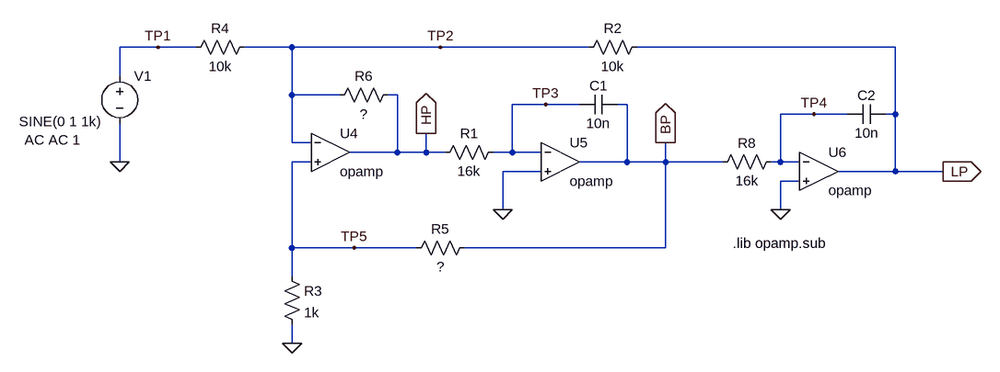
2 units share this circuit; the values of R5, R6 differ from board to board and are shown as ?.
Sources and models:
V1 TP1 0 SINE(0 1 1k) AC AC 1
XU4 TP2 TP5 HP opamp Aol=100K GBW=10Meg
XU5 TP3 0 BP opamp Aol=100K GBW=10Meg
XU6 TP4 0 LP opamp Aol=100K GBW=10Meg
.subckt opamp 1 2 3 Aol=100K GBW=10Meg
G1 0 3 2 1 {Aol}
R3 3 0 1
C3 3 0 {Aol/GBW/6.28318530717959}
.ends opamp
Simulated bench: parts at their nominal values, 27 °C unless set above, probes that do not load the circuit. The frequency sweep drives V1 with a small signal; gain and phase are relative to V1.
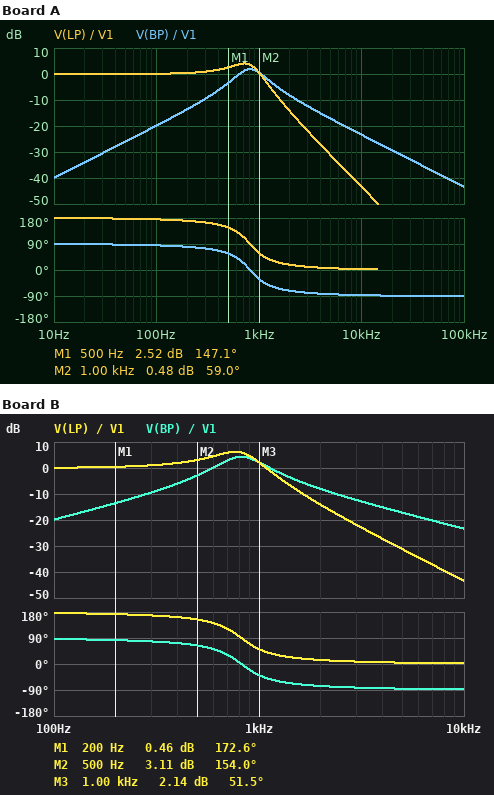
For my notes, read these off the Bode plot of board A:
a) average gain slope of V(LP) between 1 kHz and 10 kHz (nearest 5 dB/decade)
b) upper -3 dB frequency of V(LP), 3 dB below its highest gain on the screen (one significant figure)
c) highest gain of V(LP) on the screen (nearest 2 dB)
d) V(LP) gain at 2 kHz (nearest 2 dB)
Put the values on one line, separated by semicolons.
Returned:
-45 dB/decade; 1 kHz; 4 dB; -14 dB
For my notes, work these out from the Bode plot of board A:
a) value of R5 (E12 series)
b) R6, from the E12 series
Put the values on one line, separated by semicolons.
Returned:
3.3 kΩ; 6.8 kΩ
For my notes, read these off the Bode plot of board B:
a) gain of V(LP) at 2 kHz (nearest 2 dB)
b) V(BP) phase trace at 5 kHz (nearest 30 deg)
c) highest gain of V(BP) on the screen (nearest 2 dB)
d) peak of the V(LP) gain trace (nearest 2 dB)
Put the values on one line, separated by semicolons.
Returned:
-14 dB; -90 deg; 4 dB; 6 dB
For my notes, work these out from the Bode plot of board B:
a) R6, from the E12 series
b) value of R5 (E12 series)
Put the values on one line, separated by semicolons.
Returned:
6.8 kΩ; 4.7 kΩ
